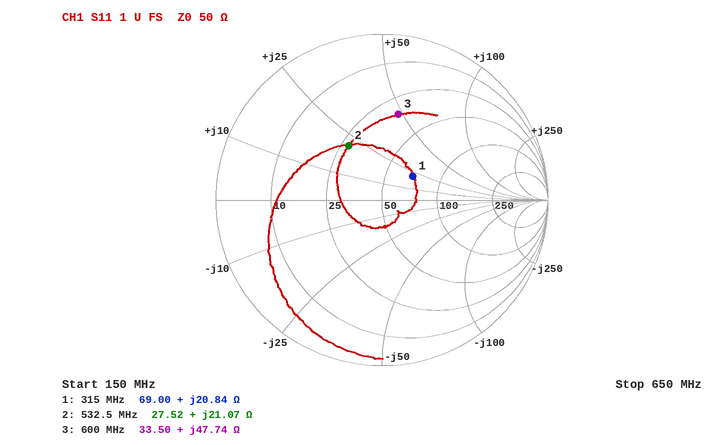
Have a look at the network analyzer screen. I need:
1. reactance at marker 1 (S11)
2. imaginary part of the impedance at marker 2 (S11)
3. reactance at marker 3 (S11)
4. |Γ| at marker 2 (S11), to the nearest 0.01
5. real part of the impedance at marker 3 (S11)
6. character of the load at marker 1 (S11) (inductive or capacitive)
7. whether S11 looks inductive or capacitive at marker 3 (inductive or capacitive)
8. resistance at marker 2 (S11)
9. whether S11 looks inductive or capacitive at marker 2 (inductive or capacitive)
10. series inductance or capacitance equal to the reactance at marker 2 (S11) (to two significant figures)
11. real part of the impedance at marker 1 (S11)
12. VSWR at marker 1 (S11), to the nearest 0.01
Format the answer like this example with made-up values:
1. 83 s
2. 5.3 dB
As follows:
1. +20.84 Ω
2. +21.07 Ω
3. +47.74 Ω
4. 0.38
5. 33.50 Ω
6. inductive
7. inductive
8. 27.52 Ω
9. inductive
10. 6.3 nH
11. 69.00 Ω
12. 1.61
